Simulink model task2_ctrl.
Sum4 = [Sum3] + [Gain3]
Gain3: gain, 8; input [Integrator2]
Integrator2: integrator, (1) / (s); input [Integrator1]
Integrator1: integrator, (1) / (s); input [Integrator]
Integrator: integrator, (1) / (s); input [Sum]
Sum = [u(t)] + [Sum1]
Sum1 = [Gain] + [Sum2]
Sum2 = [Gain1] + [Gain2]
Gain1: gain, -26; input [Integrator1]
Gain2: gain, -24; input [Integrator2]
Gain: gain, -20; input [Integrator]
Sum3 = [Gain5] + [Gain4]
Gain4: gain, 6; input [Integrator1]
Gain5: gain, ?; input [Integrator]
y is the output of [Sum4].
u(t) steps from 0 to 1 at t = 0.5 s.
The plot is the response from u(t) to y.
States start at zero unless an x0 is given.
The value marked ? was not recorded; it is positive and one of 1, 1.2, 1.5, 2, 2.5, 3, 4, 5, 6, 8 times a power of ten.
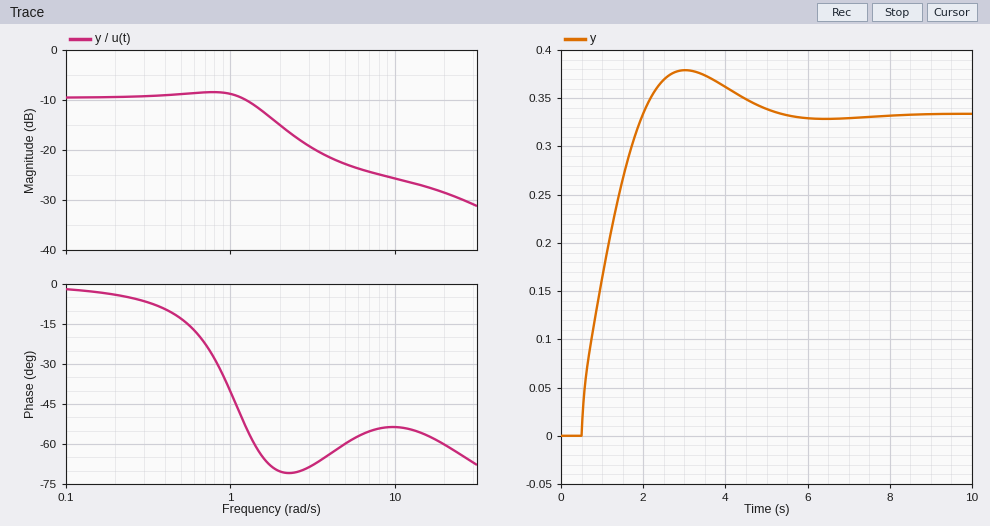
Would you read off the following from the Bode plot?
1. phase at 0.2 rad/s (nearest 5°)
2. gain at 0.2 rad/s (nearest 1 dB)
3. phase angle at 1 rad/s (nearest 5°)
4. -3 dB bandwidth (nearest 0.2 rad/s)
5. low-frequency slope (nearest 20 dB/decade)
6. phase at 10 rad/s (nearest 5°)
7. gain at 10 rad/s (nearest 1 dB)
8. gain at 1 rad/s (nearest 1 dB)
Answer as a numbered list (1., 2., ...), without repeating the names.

1. -5°
2. -9 dB
3. -40°
4. 1.6 rad/s
5. 0 dB/decade
6. -55°
7. -26 dB
8. -9 dB
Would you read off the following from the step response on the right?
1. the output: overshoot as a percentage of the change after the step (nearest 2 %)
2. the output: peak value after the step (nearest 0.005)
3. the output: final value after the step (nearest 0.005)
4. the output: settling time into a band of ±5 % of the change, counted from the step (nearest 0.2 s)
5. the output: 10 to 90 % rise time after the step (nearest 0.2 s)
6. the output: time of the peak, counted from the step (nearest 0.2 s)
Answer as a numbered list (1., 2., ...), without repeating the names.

1. 14 %
2. 0.380
3. 0.335
4. 4.0 s
5. 1.2 s
6. 2.6 s
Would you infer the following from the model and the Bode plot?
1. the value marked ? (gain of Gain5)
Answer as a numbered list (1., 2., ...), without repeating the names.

1. 1
